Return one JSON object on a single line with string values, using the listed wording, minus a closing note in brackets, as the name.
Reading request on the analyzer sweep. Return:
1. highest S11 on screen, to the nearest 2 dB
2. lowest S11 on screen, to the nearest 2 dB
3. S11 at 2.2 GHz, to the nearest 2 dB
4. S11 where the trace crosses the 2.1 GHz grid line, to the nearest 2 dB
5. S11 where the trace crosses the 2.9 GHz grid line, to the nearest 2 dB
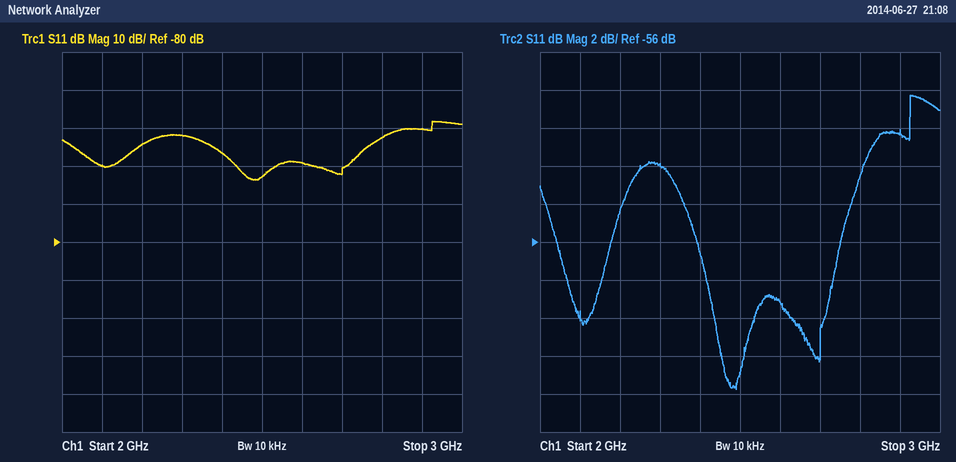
{"highest S11 on screen, to the nearest 2 dB": "-48 dB", "lowest S11 on screen, to the nearest 2 dB": "-64 dB", "S11 at 2.2 GHz, to the nearest 2 dB": "-54 dB", "S11 where the trace crosses the 2.1 GHz grid line, to the nearest 2 dB": "-60 dB", "S11 where the trace crosses the 2.9 GHz grid line, to the nearest 2 dB": "-50 dB"}
